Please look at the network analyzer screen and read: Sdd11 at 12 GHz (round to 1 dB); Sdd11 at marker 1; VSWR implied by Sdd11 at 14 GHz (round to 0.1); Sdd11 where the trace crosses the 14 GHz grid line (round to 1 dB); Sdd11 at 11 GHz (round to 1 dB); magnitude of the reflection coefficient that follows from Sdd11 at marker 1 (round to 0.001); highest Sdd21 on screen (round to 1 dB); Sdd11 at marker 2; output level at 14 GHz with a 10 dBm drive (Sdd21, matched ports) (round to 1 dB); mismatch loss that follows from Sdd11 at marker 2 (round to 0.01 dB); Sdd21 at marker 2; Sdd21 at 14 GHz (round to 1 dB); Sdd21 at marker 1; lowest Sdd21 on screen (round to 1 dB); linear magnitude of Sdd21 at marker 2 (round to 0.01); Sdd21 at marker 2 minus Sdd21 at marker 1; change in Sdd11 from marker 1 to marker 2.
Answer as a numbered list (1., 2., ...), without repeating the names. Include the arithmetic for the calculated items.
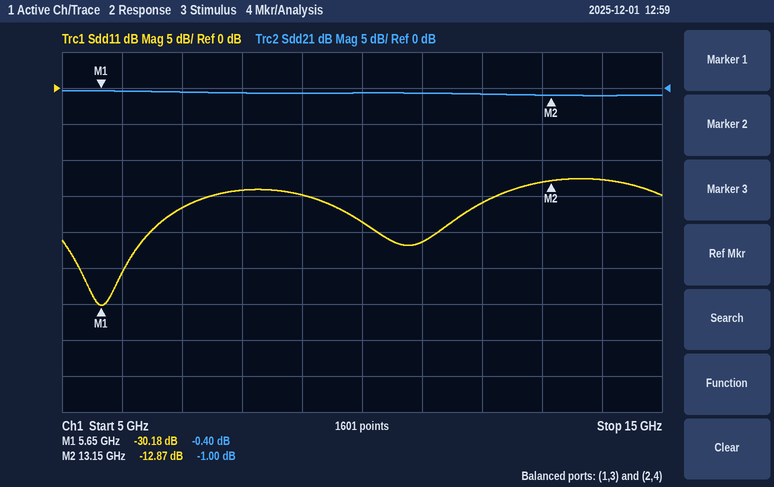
1. -16 dB
2. -30.18 dB
3. |Γ| = 10^(-13/20) = 0.2239; VSWR = (1 + 0.2239)/(1 − 0.2239) ≈ 1.6
4. -13 dB
5. -21 dB
6. 10^(-30.18/20) ≈ 0.031
7. 0 dB
8. -12.87 dB
9. 10 dBm + (-1 dB) = 9 dBm
10. −10 log10(1 − 10^(-12.87/10)) ≈ 0.23 dB
11. -1.00 dB
12. -1 dB
13. -0.40 dB
14. -1 dB
15. 10^(-1/20) ≈ 0.89
16. -1 − (-0.4) = -0.60 dB
17. -12.87 − (-30.18) = 17.31 dB
